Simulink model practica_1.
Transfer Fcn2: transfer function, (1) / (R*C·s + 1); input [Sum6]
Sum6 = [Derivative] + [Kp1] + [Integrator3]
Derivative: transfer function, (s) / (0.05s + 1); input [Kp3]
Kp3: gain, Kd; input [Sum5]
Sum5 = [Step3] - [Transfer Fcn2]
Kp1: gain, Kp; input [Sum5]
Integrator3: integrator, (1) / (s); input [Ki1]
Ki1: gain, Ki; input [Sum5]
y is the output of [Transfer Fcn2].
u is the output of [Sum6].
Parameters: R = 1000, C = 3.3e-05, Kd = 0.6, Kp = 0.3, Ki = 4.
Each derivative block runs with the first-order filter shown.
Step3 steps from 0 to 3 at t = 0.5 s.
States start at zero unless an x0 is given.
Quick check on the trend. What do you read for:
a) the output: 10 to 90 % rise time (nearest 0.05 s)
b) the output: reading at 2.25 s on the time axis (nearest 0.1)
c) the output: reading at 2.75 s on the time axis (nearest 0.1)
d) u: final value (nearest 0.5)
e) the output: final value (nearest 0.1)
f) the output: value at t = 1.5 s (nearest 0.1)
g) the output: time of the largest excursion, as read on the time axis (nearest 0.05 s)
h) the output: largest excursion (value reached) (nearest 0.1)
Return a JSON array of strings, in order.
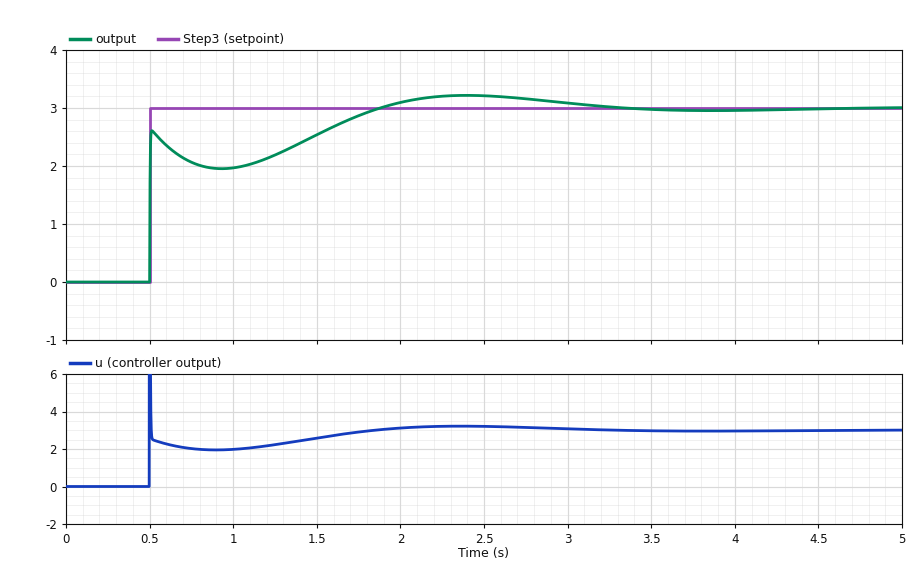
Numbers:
["1.10 s", "3.2", "3.2", "3.0", "3.0", "2.5", "2.40 s", "3.2"]
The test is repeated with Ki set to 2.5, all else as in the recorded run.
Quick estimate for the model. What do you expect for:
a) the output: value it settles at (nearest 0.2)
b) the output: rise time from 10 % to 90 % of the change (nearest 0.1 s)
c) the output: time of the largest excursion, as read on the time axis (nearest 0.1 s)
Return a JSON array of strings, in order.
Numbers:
["3.0", "1.5 s", "3.0 s"]
